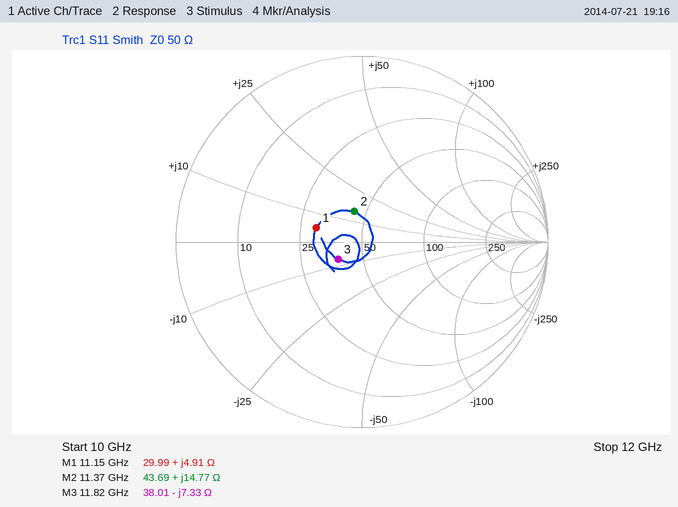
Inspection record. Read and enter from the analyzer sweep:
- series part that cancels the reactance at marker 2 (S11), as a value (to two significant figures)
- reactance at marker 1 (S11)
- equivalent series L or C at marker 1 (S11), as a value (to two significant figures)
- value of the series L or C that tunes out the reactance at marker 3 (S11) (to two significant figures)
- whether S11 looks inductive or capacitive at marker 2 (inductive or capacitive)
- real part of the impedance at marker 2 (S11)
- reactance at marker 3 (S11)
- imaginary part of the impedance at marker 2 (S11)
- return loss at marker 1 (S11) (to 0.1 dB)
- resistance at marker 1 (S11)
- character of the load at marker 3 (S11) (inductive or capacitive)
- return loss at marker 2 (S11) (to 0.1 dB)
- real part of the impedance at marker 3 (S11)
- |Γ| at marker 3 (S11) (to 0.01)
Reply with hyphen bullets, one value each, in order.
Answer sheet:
- 950 fF
- +4.91 Ω
- 70 pH
- 99 pH
- inductive
- 43.69 Ω
- -7.33 Ω
- +14.77 Ω
- 11.8 dB
- 29.99 Ω
- capacitive
- 15.4 dB
- 38.01 Ω
- 0.16
